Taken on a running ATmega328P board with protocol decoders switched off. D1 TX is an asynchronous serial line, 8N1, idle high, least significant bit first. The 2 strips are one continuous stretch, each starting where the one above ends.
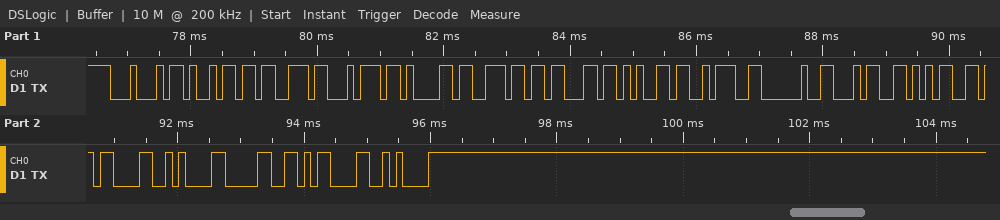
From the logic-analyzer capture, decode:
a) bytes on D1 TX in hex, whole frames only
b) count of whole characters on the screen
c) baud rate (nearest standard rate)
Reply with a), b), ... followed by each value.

a) 44 69 73 74 61 6E 63 65 3A 20 34 35 0D 0A 30 0D 0A
b) 17
c) 9600 baud
